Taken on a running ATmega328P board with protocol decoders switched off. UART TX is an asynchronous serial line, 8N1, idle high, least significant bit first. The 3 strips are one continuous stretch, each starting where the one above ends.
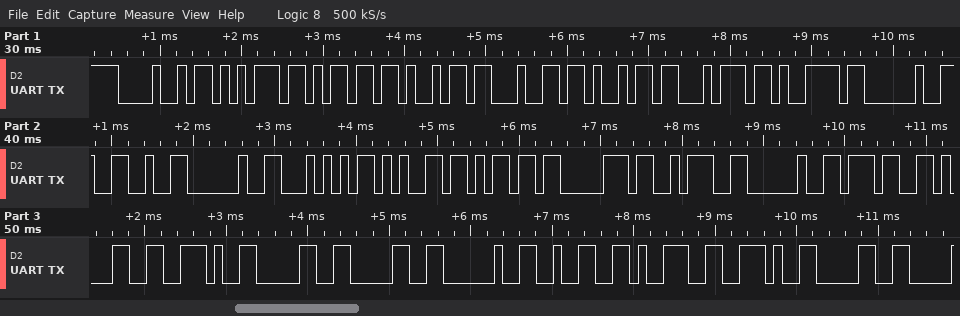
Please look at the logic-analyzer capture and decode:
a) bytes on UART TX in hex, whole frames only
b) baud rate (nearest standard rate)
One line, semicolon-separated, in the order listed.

48 75 6D 69 64 69 74 79 20 26 20 54 65 6D 70 3A 20 37 31 2E 30 30 20 32 39 2E 30; 9600 baud
